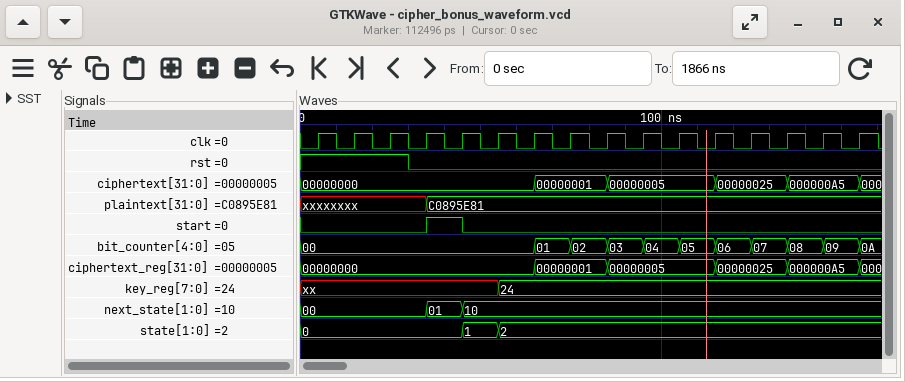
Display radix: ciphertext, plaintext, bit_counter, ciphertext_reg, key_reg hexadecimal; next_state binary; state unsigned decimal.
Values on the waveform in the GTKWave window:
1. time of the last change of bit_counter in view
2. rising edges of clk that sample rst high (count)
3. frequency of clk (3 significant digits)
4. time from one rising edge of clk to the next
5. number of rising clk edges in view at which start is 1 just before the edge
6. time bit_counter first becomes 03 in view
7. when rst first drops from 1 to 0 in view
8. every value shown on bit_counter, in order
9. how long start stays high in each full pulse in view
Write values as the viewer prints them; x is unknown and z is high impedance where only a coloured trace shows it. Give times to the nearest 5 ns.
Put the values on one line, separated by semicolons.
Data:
155 ns; 3; 100 MHz; 10 ns; 1; 85 ns; 30 ns; 00, 01, 02, 03, 04, 05, 06, 07, 08, 09, 0A; 10 ns
